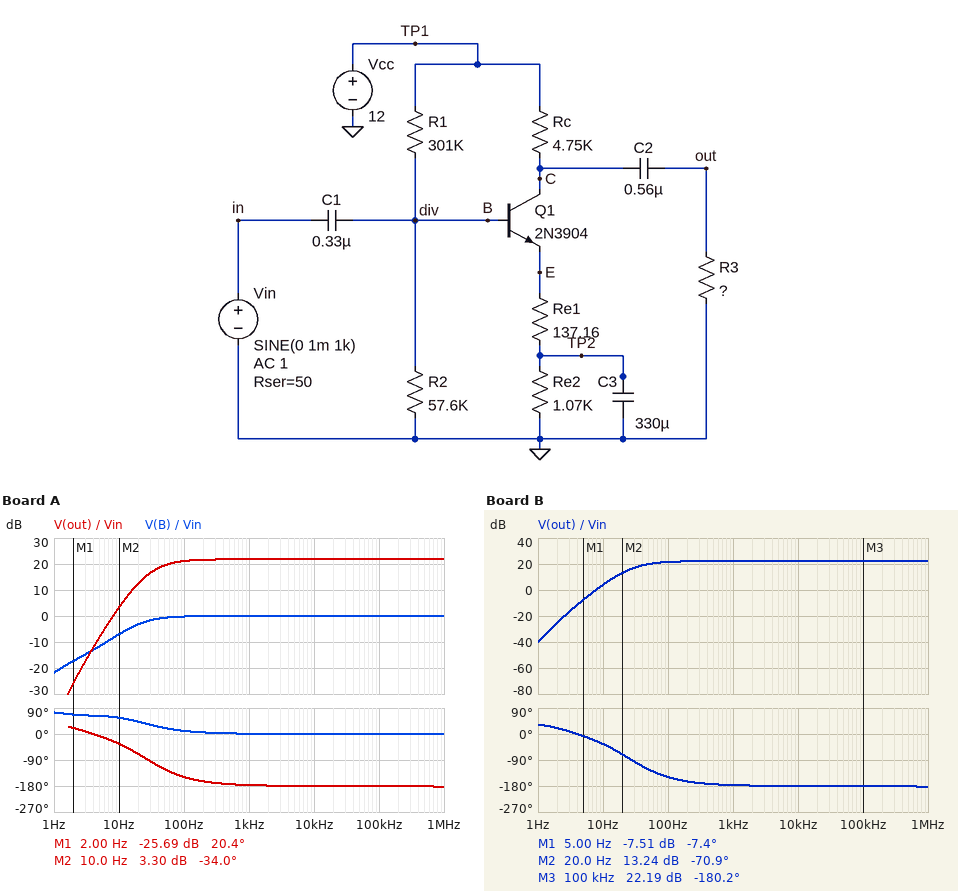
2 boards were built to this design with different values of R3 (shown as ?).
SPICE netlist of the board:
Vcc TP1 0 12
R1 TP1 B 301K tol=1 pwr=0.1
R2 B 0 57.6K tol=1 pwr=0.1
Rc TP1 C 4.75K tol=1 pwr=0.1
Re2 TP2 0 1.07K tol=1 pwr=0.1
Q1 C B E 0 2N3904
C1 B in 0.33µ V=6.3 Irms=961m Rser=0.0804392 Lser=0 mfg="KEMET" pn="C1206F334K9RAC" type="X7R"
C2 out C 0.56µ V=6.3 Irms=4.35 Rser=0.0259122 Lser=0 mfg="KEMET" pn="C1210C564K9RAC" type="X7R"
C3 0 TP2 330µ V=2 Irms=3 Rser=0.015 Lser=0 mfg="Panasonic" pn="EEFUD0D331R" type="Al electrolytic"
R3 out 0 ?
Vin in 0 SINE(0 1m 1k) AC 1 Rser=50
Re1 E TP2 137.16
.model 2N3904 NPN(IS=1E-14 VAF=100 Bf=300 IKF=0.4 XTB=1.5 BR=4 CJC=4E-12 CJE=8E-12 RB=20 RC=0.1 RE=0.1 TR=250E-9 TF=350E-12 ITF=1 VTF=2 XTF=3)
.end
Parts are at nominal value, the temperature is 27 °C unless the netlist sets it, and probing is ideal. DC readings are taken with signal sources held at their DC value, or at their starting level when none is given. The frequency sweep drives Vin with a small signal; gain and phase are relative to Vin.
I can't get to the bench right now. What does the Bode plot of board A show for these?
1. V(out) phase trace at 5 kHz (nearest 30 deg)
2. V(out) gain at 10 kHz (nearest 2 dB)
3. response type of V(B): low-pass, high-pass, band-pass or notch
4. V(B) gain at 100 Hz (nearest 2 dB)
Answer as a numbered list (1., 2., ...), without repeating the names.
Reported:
1. -180 deg
2. 22 dB
3. high-pass
4. 0 dB
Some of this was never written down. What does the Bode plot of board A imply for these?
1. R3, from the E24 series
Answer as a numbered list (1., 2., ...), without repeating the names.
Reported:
1. 3.6 kΩ
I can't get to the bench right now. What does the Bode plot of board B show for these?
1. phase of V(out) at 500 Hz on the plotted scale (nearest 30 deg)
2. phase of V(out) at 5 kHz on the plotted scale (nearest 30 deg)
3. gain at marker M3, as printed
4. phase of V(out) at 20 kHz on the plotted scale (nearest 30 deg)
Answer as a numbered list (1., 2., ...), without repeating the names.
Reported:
1. -180 deg
2. -180 deg
3. 22.19 dB
4. -180 deg
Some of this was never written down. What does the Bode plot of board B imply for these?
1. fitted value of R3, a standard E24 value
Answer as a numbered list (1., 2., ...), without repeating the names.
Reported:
1. 3.9 kΩ
